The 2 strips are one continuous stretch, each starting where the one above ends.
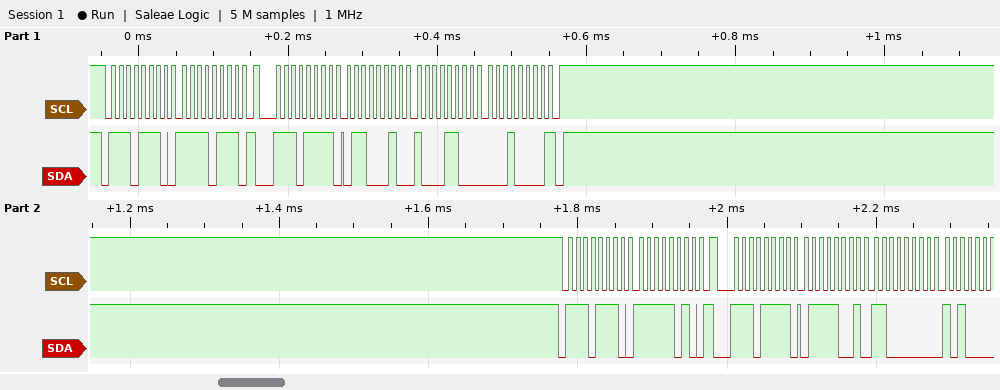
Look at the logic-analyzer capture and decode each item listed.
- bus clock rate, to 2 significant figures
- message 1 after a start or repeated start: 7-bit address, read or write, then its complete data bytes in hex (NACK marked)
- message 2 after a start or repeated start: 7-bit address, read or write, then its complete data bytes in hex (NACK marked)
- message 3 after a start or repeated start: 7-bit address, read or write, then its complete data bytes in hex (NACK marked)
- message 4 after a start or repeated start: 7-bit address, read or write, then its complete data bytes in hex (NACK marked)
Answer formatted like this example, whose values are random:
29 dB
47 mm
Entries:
100 kHz
0x77 write: F7
0x77 read: 62 8C 10 NACK
0x77 write: FA
0x77 read: 79 C0
